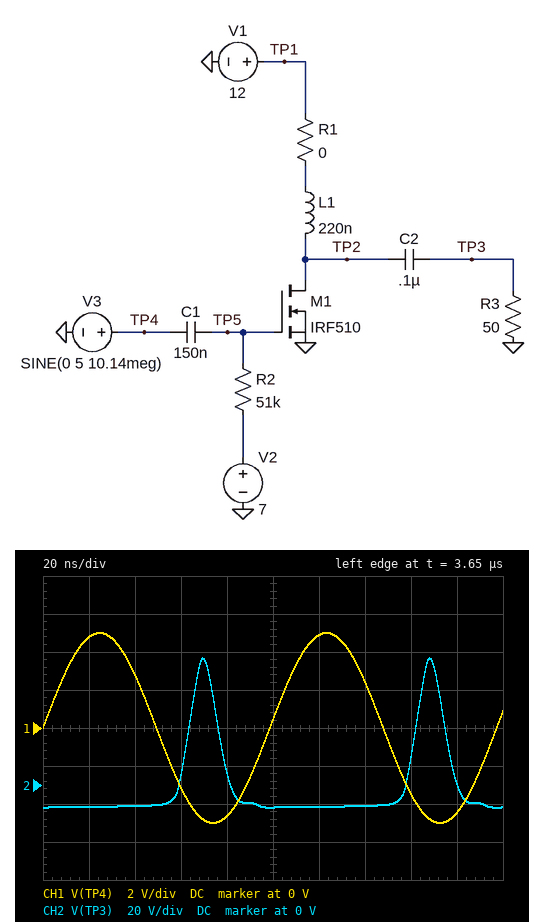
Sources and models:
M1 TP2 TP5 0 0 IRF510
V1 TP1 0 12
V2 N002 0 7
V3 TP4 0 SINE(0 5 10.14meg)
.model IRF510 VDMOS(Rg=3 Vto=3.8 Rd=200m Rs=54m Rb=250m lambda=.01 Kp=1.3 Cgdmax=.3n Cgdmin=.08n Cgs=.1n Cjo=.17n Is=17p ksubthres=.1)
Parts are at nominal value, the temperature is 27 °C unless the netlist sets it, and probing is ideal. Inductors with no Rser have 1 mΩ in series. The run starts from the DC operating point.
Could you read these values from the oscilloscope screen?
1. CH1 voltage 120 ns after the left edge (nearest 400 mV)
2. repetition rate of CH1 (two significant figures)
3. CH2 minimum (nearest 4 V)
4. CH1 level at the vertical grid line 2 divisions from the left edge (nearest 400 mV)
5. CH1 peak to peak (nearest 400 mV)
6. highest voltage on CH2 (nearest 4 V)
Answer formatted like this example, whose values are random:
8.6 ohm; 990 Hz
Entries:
4.8 V; 10 MHz; -12 V; 2.8 V; 10.0 V; 68 V
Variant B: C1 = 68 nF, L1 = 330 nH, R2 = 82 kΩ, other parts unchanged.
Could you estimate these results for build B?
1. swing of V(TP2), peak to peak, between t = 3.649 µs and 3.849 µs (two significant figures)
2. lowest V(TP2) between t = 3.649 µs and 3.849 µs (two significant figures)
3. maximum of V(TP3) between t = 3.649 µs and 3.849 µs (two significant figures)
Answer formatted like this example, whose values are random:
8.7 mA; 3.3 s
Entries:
65 V; 180 mV; 53 V
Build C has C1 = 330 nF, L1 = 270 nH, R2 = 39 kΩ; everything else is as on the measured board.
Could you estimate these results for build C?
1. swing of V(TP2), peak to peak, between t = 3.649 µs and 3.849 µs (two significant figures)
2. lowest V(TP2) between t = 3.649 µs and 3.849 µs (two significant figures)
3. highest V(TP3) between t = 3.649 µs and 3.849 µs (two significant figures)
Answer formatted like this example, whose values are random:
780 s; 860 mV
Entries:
72 V; 210 mV; 60 V
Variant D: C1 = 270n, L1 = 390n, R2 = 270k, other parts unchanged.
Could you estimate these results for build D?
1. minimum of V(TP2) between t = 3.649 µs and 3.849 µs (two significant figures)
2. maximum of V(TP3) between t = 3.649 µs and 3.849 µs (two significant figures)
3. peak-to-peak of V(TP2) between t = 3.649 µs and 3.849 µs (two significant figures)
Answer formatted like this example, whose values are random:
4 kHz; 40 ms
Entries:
170 mV; 48 V; 60 V
